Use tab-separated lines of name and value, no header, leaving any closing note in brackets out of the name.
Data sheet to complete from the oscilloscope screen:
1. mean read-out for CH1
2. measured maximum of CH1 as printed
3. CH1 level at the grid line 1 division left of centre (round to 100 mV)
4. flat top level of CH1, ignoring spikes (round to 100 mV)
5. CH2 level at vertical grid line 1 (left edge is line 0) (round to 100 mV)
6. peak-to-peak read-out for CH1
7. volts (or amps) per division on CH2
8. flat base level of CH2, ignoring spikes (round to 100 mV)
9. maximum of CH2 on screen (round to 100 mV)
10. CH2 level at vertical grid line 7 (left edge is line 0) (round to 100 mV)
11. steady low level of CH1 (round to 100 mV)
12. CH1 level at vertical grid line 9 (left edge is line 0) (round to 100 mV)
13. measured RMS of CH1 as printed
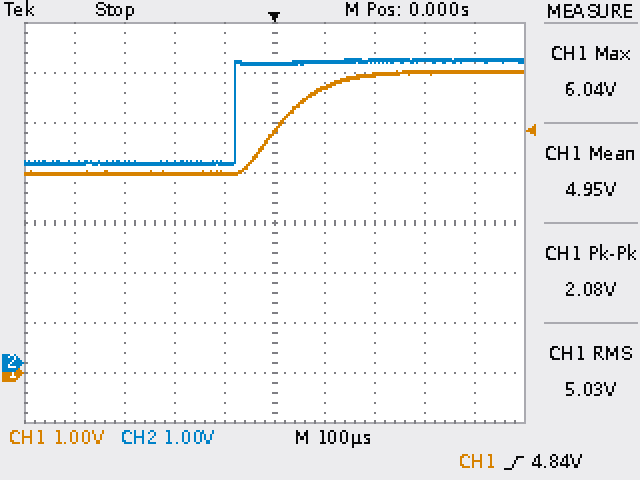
mean read-out for CH1	4.95 V
measured maximum of CH1 as printed	6.04 V
CH1 level at the grid line 1 division left of centre	4.0 V
flat top level of CH1, ignoring spikes	6.0 V
CH2 level at vertical grid line 1 (left edge is line 0)	4.0 V
peak-to-peak read-out for CH1	2.08 V
volts (or amps) per division on CH2	1 V
flat base level of CH2, ignoring spikes	4.0 V
maximum of CH2 on screen	6.1 V
CH2 level at vertical grid line 7 (left edge is line 0)	6.0 V
steady low level of CH1	4.0 V
CH1 level at vertical grid line 9 (left edge is line 0)	6.0 V
measured RMS of CH1 as printed	5.03 V
